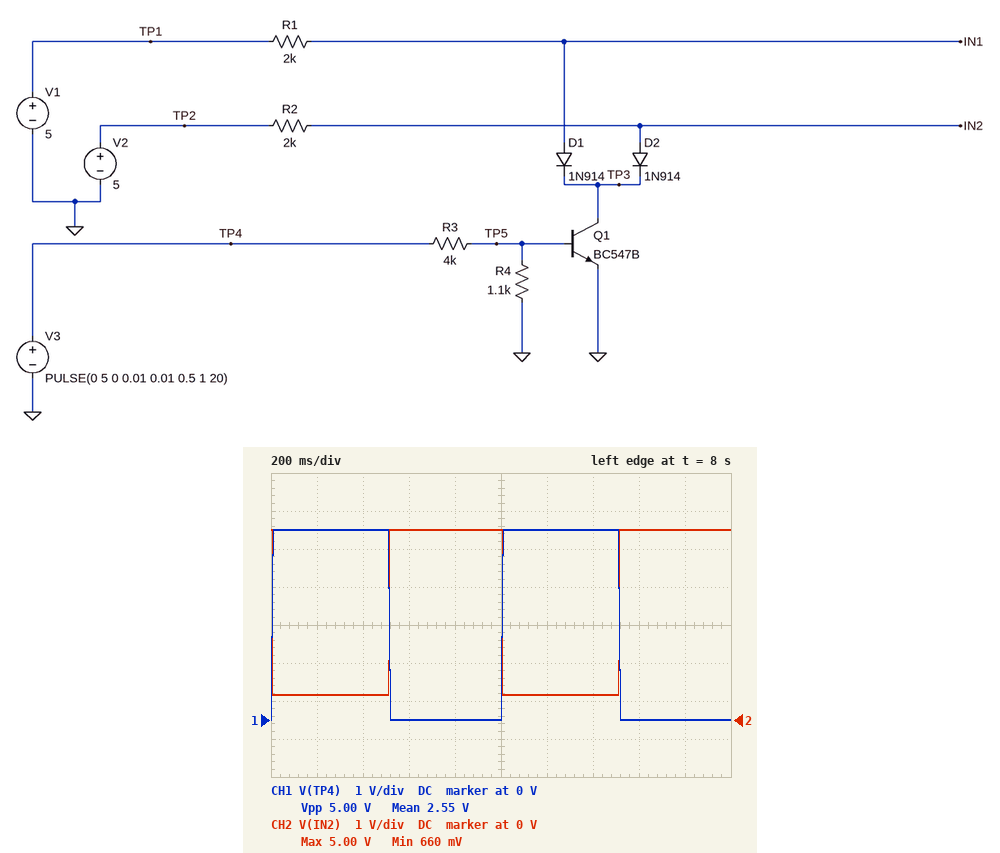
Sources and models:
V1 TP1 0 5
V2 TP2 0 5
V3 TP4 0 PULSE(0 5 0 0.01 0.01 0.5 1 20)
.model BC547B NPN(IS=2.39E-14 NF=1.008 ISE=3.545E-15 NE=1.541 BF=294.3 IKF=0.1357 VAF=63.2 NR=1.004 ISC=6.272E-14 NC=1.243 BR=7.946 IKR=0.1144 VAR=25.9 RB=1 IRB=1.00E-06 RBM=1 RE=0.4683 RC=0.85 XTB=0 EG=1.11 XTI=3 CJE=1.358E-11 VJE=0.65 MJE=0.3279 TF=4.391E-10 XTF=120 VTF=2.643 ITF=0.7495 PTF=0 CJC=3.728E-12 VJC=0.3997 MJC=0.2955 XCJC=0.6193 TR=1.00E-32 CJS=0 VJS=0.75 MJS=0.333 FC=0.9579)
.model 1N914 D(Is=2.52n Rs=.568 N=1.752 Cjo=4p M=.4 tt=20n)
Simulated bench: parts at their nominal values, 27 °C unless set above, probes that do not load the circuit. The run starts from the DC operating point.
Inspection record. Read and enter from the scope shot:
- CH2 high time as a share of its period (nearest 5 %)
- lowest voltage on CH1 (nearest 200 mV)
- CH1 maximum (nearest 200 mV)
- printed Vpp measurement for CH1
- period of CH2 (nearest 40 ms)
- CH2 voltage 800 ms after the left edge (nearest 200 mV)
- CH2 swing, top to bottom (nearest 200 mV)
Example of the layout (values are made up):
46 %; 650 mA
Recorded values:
50 %; 0 V; 5.0 V; 5.00 V; 1.00 s; 5.0 V; 4.4 V
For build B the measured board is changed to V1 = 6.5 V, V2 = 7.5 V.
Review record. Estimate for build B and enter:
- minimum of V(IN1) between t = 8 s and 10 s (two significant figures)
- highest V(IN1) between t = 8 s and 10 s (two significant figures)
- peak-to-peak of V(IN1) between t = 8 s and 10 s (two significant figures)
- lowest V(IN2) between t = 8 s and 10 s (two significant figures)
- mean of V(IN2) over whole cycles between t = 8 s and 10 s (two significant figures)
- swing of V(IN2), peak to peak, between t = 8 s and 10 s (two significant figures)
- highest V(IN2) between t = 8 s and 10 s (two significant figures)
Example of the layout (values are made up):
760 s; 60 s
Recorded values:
680 mV; 6.5 V; 5.8 V; 690 mV; 4.0 V; 6.8 V; 7.5 V
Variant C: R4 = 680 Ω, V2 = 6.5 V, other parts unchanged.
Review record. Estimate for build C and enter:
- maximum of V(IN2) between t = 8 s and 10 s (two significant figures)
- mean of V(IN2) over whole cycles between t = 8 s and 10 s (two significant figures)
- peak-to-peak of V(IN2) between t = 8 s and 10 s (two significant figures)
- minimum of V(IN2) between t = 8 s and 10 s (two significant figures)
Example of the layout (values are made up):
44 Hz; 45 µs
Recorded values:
6.5 V; 3.6 V; 5.8 V; 720 mV
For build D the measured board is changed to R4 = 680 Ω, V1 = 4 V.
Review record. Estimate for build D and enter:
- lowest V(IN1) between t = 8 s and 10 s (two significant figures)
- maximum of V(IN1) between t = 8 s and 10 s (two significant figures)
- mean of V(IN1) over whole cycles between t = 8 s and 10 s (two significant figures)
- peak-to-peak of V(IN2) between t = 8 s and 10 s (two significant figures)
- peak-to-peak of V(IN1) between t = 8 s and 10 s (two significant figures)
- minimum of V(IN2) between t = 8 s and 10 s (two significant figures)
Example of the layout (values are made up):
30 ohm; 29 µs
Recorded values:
680 mV; 4.0 V; 2.3 V; 4.3 V; 3.3 V; 690 mV
